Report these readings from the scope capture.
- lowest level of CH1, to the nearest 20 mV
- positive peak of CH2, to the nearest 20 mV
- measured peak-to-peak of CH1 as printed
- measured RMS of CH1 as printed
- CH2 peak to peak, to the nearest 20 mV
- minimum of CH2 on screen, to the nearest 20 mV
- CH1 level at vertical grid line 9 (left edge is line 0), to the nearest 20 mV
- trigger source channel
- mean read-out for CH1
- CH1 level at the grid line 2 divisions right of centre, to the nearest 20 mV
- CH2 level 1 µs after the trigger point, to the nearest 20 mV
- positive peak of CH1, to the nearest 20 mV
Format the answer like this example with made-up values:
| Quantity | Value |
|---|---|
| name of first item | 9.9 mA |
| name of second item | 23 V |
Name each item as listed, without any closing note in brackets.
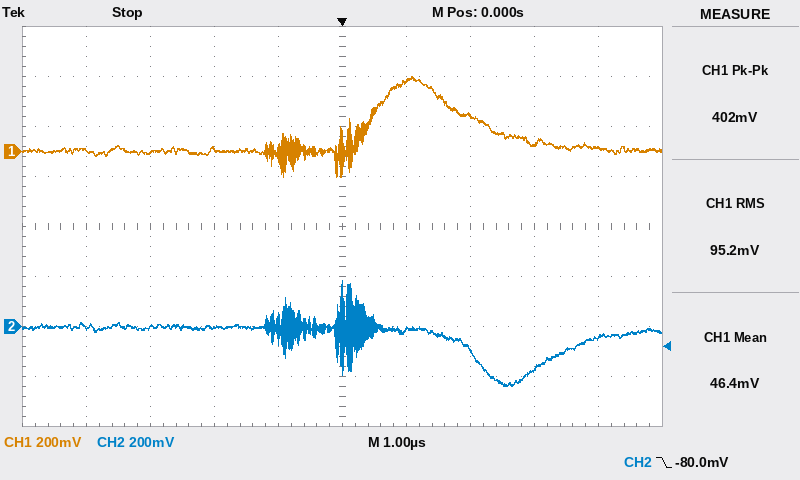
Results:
| Quantity | Value |
|---|---|
| lowest level of CH1, to the nearest 20 mV | -100 mV |
| positive peak of CH2, to the nearest 20 mV | 180 mV |
| measured peak-to-peak of CH1 as printed | 402 mV |
| measured RMS of CH1 as printed | 95.2 mV |
| CH2 peak to peak, to the nearest 20 mV | 420 mV |
| minimum of CH2 on screen, to the nearest 20 mV | -240 mV |
| CH1 level at vertical grid line 9 (left edge is line 0), to the nearest 20 mV | 20 mV |
| trigger source channel | CH2 |
| mean read-out for CH1 | 46.4 mV |
| CH1 level at the grid line 2 divisions right of centre, to the nearest 20 mV | 140 mV |
| CH2 level 1 µs after the trigger point, to the nearest 20 mV | -20 mV |
| positive peak of CH1, to the nearest 20 mV | 300 mV |
